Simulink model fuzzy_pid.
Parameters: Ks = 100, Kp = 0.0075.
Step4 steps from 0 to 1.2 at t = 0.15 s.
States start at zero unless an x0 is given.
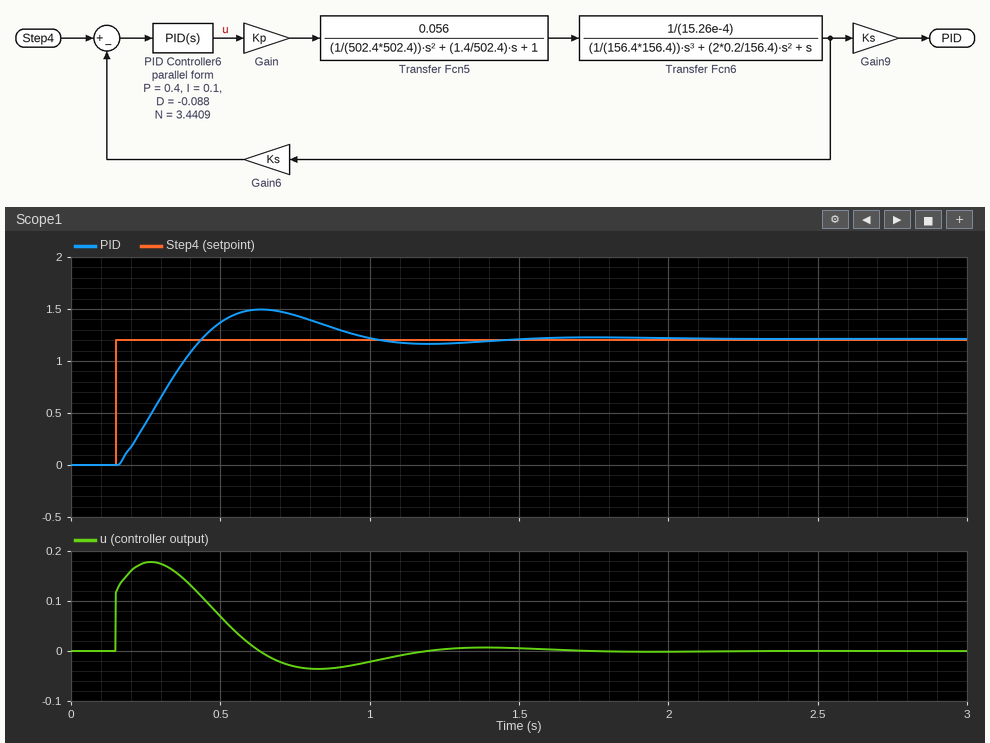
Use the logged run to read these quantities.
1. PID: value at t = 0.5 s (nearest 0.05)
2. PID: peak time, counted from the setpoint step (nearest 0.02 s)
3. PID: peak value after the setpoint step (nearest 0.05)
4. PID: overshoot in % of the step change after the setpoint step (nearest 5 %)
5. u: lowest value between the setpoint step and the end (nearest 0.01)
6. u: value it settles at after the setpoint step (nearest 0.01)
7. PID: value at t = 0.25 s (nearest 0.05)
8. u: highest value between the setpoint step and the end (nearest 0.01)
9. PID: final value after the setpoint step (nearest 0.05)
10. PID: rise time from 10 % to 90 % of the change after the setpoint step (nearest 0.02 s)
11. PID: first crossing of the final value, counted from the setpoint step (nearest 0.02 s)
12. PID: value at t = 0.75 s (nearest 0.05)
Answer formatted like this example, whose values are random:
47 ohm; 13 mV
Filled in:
1.35; 0.48 s; 1.50; 25 %; -0.04; 0.00; 0.40; 0.18; 1.20; 0.22 s; 0.28 s; 1.45
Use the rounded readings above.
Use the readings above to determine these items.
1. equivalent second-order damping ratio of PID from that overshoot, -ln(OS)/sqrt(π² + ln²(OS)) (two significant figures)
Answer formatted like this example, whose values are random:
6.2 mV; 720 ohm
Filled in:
0.40
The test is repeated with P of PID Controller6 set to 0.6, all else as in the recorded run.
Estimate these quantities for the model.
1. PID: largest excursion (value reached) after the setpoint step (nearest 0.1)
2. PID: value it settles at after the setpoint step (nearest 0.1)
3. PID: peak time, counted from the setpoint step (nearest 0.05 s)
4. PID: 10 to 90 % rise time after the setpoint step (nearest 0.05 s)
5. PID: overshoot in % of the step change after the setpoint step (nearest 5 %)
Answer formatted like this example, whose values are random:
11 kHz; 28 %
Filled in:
1.3; 1.2; 0.35 s; 0.15 s; 10 %
